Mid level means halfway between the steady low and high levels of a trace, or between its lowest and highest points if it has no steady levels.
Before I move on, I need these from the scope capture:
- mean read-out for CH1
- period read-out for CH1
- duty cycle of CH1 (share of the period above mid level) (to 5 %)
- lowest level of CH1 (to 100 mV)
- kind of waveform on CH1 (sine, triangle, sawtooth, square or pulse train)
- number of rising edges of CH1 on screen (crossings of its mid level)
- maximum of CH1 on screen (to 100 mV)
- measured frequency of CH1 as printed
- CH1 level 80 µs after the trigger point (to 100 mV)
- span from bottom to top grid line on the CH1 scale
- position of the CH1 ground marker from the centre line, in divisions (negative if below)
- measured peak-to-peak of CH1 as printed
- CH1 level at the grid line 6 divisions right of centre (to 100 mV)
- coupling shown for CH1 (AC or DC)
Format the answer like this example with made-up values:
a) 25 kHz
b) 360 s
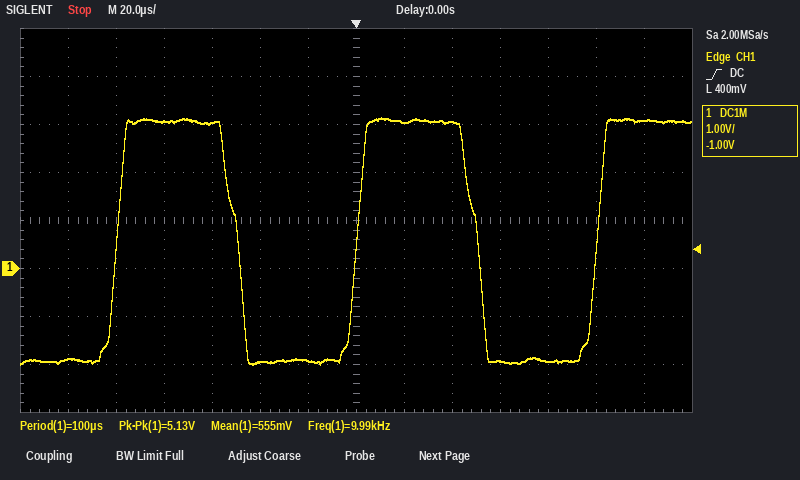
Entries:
a) 555 mV
b) 100 µs
c) 50 %
d) -2.0 V
e) square
f) 3
g) 3.1 V
h) 9.99 kHz
i) -1.9 V
j) 8 V
k) -1.0 div
l) 5.13 V
m) 3.1 V
n) DC
